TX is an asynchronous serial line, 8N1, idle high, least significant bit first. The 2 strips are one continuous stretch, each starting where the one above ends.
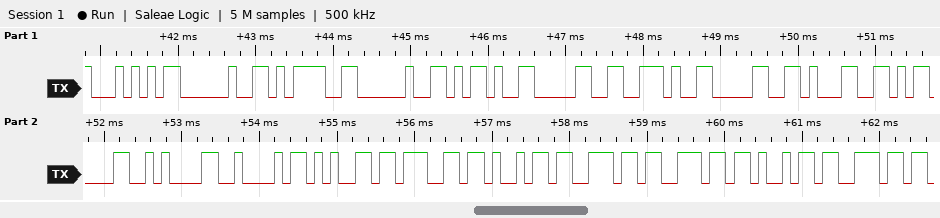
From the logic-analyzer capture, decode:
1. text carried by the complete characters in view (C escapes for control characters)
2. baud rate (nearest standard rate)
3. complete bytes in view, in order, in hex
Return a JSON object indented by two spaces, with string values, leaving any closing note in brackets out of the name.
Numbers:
{
  "text carried by the complete characters in view": "\"T = -0.01\\r\\nBeginnin\"",
  "baud rate": "9600 baud",
  "complete bytes in view, in order, in hex": "0x54 0x20 0x3D 0x20 0x2D 0x30 0x2E 0x30 0x31 0x0D 0x0A 0x42 0x65 0x67 0x69 0x6E 0x6E 0x69 0x6E"
}
